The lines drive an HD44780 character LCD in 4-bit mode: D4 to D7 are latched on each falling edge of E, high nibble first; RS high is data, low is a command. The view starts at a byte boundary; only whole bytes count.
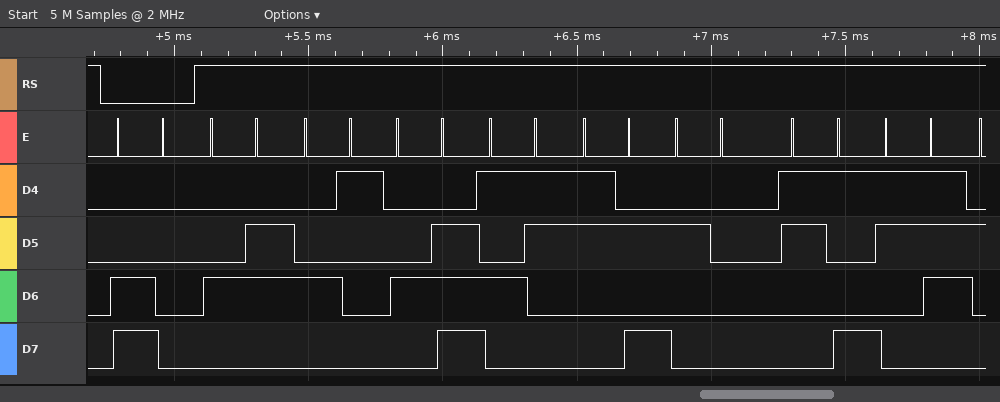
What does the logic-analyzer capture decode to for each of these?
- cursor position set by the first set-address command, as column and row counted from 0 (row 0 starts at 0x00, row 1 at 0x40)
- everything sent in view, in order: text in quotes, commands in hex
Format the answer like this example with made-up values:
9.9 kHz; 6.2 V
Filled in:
column 0, row 1; 0xC0 "FANS: 97"
